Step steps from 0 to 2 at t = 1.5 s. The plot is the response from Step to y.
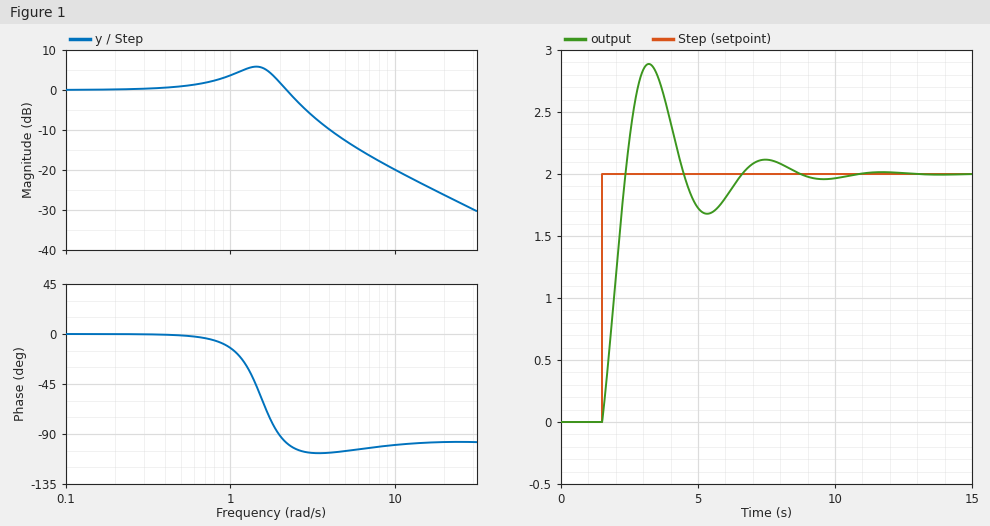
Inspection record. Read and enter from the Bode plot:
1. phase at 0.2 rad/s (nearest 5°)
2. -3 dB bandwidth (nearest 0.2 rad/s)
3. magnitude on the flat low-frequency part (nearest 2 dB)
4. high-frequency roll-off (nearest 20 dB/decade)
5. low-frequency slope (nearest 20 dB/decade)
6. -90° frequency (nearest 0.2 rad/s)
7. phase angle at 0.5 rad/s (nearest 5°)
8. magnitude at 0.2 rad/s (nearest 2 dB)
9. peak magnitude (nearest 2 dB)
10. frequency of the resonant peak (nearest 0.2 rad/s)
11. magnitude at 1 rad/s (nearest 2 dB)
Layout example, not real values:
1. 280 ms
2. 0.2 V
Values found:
1. 0°
2. 2.6 rad/s
3. 0 dB
4. -20 dB/decade
5. 0 dB/decade
6. 2.0 rad/s
7. 0°
8. 0 dB
9. 6 dB
10. 1.4 rad/s
11. 4 dB
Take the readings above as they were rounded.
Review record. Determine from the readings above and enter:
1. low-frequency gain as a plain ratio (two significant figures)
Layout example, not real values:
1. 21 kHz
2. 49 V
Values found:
1. 1.0
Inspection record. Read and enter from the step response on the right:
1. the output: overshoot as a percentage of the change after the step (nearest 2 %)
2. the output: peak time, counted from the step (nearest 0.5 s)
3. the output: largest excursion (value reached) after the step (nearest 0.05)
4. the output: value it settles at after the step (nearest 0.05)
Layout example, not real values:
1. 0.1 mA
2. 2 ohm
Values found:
1. 44 %
2. 1.5 s
3. 2.90
4. 2.00
